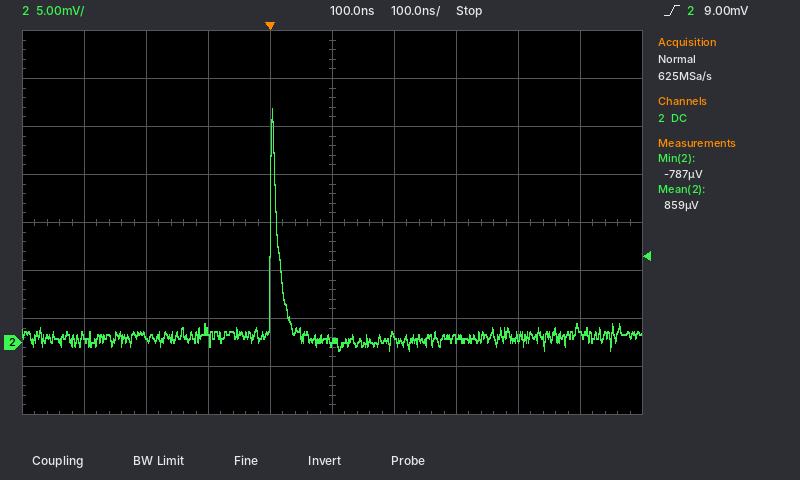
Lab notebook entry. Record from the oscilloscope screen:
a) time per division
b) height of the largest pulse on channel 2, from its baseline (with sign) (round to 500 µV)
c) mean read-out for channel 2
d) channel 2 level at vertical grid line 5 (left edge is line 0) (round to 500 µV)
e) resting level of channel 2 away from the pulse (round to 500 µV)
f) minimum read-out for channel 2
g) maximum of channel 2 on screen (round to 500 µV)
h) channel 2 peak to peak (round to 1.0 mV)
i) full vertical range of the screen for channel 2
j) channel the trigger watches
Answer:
100 ns
+24.0 mV
859 µV
0.0 mV
500 µV
-787 µV
24.5 mV
25.0 mV
40 mV
channel 2
